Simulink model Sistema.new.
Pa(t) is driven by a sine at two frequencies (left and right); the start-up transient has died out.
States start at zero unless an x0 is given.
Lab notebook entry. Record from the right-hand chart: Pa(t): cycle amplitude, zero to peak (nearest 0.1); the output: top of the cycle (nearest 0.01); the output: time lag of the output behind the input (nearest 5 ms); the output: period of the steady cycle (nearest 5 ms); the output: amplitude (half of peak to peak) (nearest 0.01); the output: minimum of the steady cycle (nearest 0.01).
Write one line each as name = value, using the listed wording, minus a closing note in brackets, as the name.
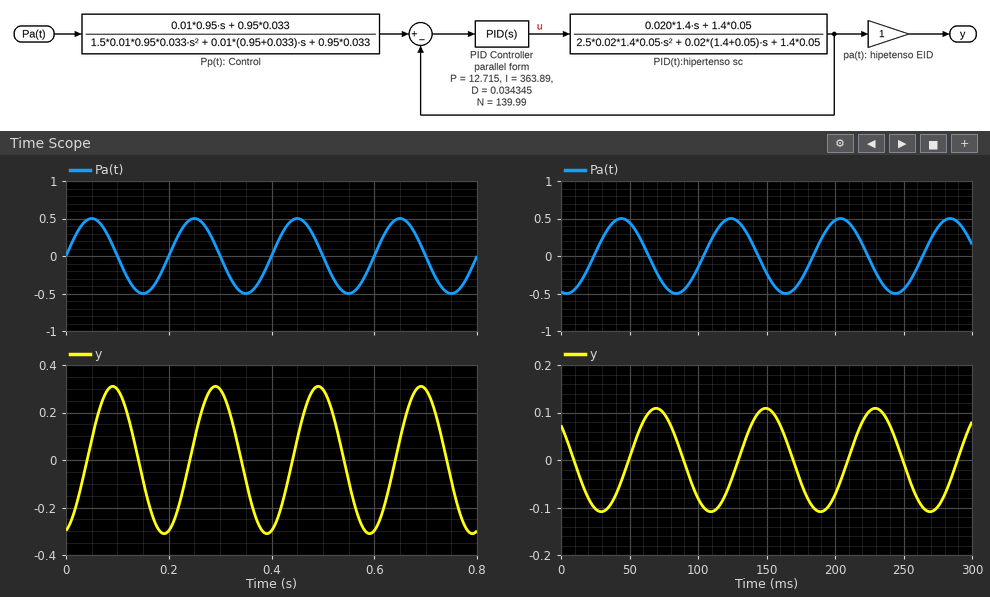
Pa(t): cycle amplitude, zero to peak = 0.5
the output: top of the cycle = 0.11
the output: time lag of the output behind the input = 25 ms
the output: period of the steady cycle = 80 ms
the output: amplitude (half of peak to peak) = 0.11
the output: minimum of the steady cycle = -0.11
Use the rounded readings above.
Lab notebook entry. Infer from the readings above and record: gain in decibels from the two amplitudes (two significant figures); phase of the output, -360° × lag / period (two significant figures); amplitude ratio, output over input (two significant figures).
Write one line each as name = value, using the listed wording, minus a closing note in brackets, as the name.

gain in decibels from the two amplitudes = -13 dB
phase of the output, -360° × lag / period = -110°
amplitude ratio, output over input = 0.22
